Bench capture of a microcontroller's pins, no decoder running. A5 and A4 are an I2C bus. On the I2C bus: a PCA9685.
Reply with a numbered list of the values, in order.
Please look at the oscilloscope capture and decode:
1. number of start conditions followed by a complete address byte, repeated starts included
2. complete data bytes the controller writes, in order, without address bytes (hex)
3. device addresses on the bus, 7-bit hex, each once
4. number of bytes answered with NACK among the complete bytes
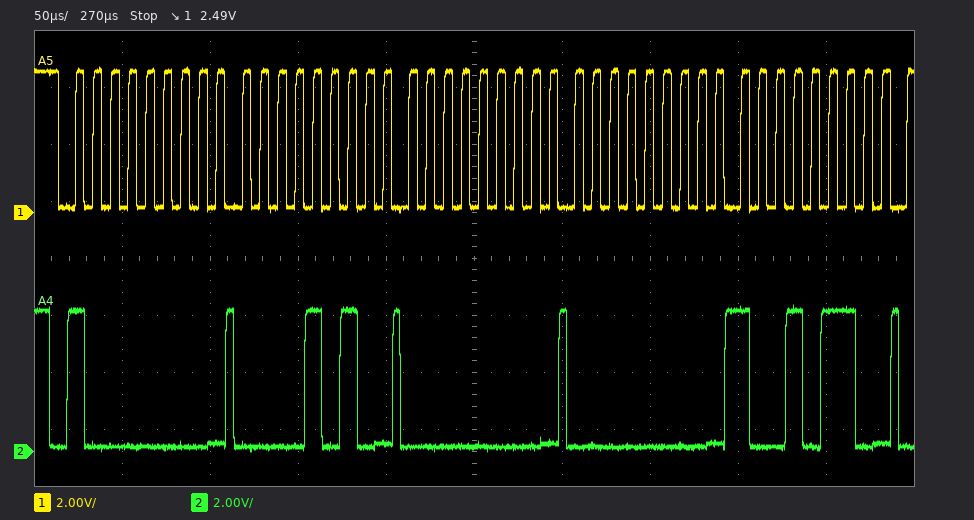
1. 1
2. 0A 00 00 96
3. 0x40
4. 0
